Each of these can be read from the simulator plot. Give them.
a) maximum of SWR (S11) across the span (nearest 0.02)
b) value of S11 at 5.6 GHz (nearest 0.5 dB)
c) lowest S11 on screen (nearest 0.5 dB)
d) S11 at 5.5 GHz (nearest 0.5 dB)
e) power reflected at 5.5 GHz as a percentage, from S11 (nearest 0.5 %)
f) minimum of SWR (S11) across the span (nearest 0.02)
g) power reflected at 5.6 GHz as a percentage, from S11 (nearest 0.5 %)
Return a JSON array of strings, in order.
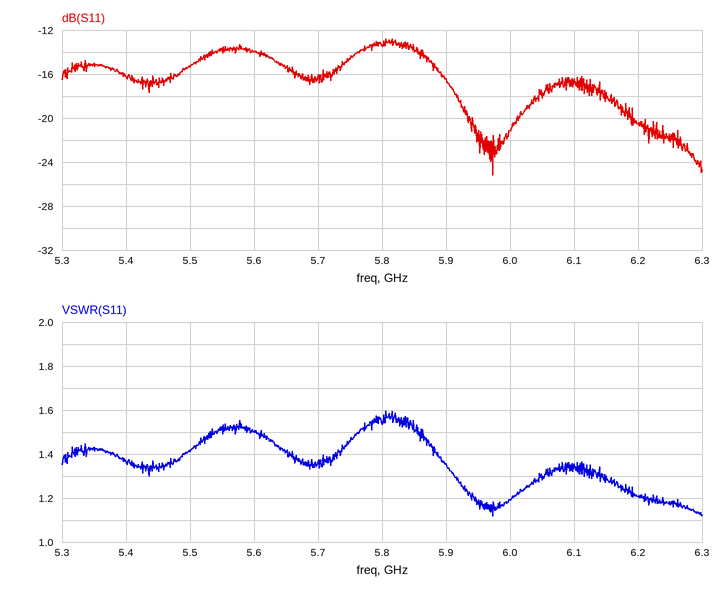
["1.60", "-14.0 dB", "-25.0 dB", "-15.5 dB", "3.0 %", "1.12", "4.0 %"]
